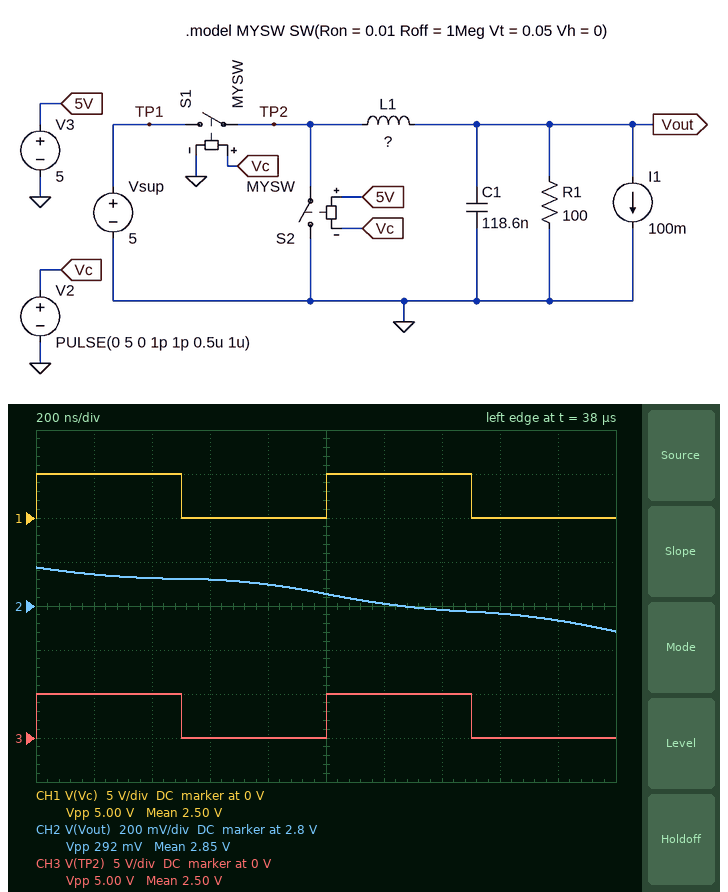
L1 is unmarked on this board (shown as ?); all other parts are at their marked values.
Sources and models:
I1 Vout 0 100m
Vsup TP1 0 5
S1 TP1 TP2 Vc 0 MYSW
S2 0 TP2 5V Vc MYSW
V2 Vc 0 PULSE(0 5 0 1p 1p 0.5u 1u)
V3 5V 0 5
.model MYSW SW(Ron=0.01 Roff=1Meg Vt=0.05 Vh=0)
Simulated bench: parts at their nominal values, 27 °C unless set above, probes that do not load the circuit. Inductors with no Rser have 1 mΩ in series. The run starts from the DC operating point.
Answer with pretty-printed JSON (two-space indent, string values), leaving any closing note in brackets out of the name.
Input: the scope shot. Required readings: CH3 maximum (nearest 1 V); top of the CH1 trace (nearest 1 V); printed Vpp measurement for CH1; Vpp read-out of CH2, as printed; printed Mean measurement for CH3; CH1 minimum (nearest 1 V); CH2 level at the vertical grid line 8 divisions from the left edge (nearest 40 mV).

{
  "CH3 maximum": "5 V",
  "top of the CH1 trace": "5 V",
  "printed Vpp measurement for CH1": "5.00 V",
  "Vpp read-out of CH2, as printed": "292 mV",
  "printed Mean measurement for CH3": "2.50 V",
  "CH1 minimum": "0 V",
  "CH2 level at the vertical grid line 8 divisions from the left edge": "2.76 V"
}
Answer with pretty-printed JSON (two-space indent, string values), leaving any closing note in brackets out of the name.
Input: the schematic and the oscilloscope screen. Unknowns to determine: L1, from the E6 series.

{
  "L1, from the E6 series": "47 µH"
}
